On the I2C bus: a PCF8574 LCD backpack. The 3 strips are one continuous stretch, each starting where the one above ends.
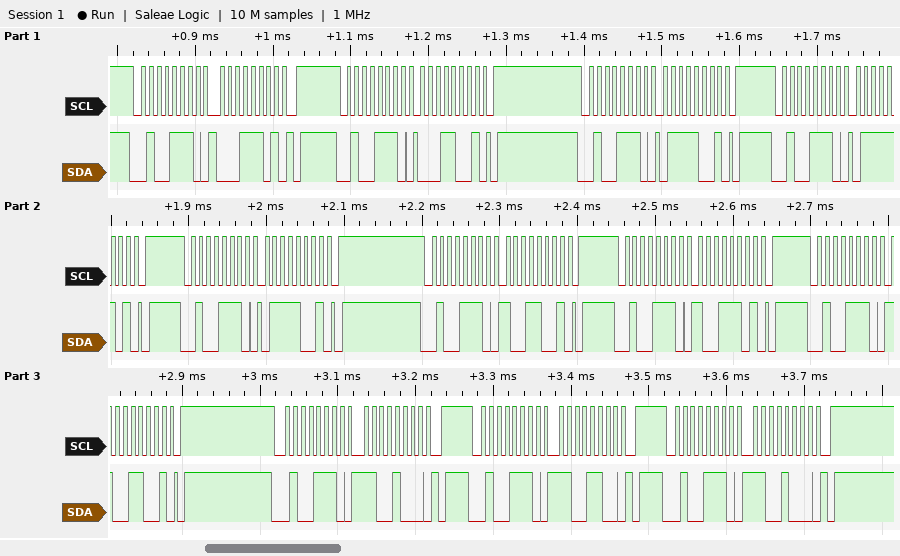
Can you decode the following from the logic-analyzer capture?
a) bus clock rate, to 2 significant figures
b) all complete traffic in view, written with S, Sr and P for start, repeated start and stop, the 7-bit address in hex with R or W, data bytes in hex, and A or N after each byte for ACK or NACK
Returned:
100 kHz
S 27W A 1D A P S 27W A 19 A P S 27W A 79 A P S 27W A 7D A P S 27W A 79 A P S 27W A 99 A P S 27W A 9D A P S 27W A 99 A P S 27W A C8 A P S 27W A CC A P S 27W A C8 A P
